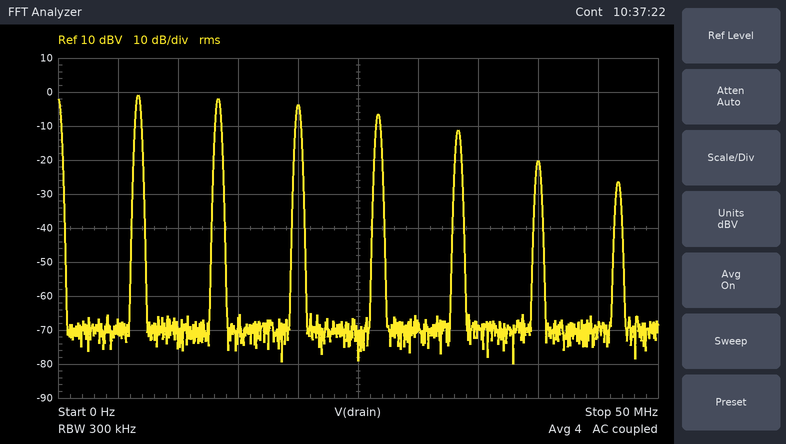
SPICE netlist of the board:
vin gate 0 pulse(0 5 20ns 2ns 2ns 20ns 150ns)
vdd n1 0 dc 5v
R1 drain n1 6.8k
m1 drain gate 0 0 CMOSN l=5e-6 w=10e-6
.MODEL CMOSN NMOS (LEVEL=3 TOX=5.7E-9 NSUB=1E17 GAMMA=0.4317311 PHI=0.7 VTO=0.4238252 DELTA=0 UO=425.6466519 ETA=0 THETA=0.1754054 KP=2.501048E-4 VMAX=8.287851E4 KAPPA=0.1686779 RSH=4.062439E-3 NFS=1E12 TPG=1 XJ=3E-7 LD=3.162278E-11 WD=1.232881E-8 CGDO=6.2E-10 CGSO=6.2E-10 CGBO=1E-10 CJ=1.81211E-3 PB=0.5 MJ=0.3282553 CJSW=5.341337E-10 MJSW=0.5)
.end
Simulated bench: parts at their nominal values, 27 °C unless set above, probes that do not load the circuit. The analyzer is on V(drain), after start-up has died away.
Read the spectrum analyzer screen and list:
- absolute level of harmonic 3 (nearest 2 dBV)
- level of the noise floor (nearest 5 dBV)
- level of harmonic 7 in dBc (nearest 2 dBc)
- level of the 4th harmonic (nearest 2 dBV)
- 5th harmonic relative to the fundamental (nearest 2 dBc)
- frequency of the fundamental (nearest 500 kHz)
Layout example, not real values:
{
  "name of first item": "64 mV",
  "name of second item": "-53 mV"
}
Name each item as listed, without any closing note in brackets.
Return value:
{
  "absolute level of harmonic 3": "-4 dBV",
  "level of the noise floor": "-70 dBV",
  "level of harmonic 7 in dBc": "-26 dBc",
  "level of the 4th harmonic": "-6 dBV",
  "5th harmonic relative to the fundamental": "-10 dBc",
  "frequency of the fundamental": "6.5 MHz"
}
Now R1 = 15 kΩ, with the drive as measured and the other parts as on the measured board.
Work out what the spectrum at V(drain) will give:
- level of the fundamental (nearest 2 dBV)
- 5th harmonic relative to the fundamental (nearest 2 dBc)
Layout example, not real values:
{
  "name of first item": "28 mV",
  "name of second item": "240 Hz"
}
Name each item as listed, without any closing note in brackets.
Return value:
{
  "level of the fundamental": "0 dBV",
  "5th harmonic relative to the fundamental": "-12 dBc"
}
